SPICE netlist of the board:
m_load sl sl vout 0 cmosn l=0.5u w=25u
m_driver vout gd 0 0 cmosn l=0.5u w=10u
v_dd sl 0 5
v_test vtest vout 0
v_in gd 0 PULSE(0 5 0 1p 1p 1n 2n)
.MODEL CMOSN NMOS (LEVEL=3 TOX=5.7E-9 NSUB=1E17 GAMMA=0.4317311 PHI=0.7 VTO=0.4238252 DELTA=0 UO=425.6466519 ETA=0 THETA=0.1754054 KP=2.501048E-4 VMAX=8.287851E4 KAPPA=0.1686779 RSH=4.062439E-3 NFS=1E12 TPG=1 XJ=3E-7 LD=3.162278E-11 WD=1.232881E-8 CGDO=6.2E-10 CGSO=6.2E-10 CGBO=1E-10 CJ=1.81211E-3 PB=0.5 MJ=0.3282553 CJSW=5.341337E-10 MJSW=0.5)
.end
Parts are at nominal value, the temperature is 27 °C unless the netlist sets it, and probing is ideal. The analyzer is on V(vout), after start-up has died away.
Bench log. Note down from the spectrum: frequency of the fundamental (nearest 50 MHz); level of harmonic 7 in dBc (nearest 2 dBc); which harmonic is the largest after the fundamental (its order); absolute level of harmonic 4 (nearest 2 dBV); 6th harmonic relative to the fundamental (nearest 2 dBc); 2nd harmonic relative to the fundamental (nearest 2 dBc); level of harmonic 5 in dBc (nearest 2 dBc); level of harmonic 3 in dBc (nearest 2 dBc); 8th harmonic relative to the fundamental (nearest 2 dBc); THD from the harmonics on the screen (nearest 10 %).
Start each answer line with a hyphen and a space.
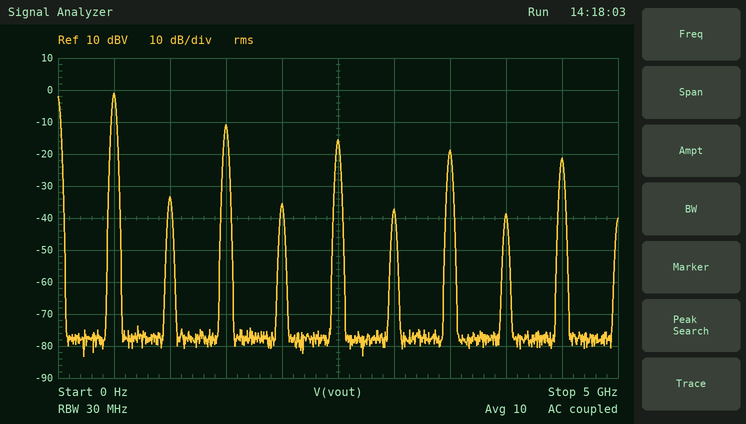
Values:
- 500 MHz
- -18 dBc
- 3
- -36 dBV
- -36 dBc
- -32 dBc
- -14 dBc
- -10 dBc
- -38 dBc
- 40 %
